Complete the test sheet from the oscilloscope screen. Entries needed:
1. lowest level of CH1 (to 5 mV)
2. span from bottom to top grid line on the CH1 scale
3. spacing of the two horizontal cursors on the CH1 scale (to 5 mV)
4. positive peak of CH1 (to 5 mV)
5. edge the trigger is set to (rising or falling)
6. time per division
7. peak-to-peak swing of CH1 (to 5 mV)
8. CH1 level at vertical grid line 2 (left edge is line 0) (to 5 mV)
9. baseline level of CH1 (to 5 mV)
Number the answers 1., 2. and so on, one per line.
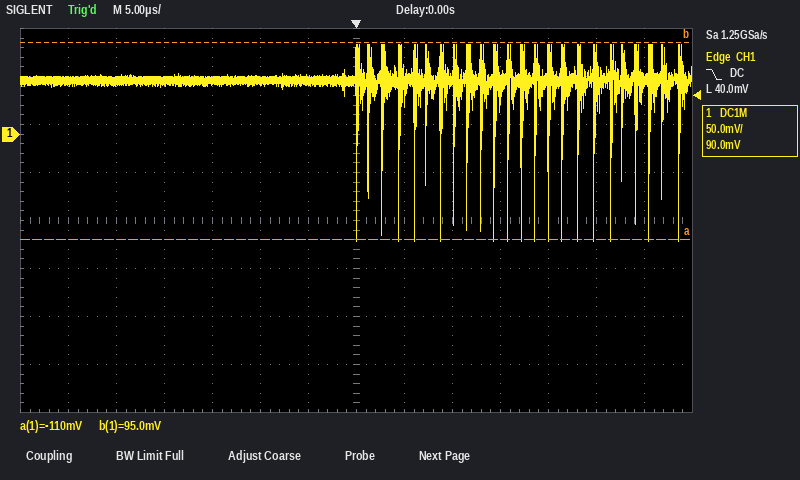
1. -110 mV
2. 400 mV
3. 205 mV
4. 95 mV
5. falling
6. 5 µs
7. 205 mV
8. 55 mV
9. 55 mV
